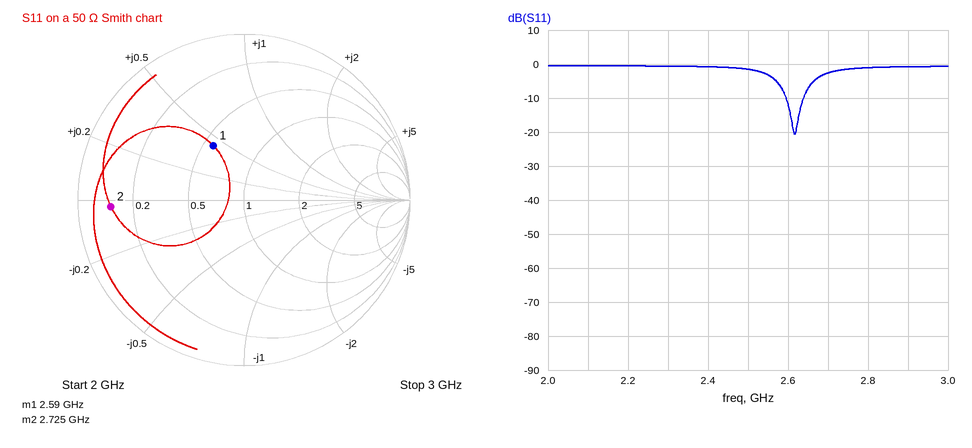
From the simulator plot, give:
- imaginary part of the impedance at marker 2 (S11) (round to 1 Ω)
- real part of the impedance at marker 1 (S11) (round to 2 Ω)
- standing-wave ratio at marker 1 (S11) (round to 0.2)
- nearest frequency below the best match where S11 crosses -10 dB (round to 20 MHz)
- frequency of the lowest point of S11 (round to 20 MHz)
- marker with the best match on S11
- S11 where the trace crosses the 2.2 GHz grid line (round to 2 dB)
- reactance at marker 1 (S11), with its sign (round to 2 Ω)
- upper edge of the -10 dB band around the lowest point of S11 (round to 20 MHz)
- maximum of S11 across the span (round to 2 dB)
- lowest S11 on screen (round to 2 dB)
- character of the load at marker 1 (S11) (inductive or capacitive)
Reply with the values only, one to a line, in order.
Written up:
-1 Ω
28 Ω
2.2
2.60 GHz
2.62 GHz
marker 1
0 dB
+22 Ω
2.64 GHz
0 dB
-20 dB
inductive
